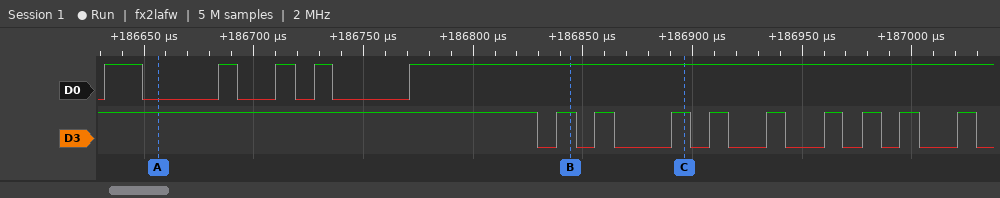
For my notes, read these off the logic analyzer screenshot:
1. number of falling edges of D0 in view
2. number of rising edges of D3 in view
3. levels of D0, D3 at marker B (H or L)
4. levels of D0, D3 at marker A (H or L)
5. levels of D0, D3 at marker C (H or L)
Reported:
4
9
D0=H, D3=H
D0=L, D3=H
D0=H, D3=H
